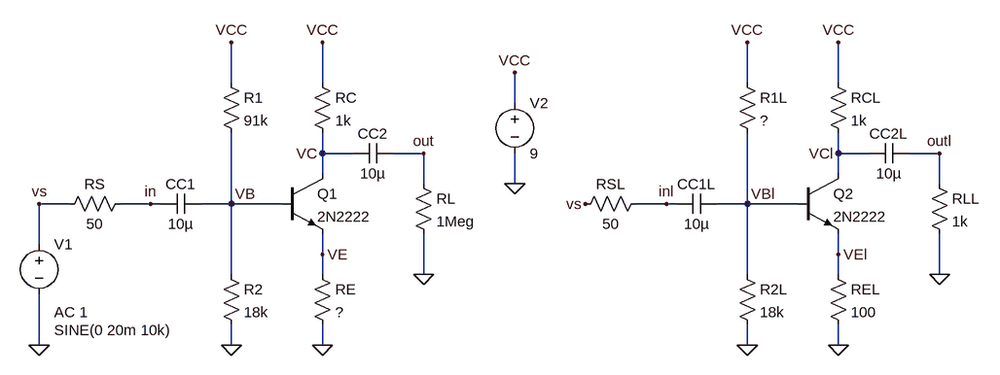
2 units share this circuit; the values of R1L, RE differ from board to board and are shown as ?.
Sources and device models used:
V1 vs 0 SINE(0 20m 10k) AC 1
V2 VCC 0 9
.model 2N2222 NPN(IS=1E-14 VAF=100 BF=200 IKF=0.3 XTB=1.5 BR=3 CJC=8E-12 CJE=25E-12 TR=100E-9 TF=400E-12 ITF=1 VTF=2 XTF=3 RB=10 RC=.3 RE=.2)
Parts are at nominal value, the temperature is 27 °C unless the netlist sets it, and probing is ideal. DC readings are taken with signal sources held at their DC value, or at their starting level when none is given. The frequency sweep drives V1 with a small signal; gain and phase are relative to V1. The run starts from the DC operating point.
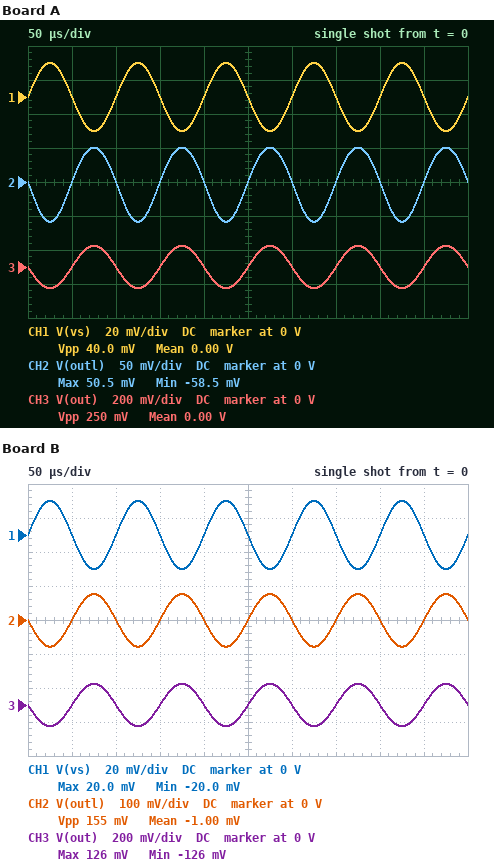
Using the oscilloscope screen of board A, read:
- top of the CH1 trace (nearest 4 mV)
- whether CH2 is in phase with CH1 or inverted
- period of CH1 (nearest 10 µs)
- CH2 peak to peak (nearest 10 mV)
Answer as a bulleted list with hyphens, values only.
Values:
- 20 mV
- inverted
- 100 µs
- 110 mV
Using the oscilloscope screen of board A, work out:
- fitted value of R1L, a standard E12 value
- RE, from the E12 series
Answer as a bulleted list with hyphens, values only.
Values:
- 220 kΩ
- 150 Ω
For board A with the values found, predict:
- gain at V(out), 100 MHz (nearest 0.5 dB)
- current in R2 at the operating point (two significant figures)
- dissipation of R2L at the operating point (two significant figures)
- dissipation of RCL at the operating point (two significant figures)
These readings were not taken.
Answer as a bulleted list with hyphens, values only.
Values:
- 5.0 dB
- 68 µA
- 24 µW
- 100 µW
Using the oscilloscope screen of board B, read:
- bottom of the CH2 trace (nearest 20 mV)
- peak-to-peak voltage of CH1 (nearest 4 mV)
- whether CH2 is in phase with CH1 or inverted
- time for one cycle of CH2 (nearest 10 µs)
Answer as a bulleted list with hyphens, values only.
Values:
- -80 mV
- 40 mV
- inverted
- 100 µs
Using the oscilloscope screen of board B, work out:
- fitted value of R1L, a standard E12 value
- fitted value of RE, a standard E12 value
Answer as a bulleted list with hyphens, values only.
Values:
- 180 kΩ
- 150 Ω
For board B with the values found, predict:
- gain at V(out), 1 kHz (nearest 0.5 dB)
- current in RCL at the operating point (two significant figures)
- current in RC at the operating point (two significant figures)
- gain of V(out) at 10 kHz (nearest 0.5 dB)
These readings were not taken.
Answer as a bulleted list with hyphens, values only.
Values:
- 16.0 dB
- 940 µA
- 3.6 mA
- 16.0 dB
